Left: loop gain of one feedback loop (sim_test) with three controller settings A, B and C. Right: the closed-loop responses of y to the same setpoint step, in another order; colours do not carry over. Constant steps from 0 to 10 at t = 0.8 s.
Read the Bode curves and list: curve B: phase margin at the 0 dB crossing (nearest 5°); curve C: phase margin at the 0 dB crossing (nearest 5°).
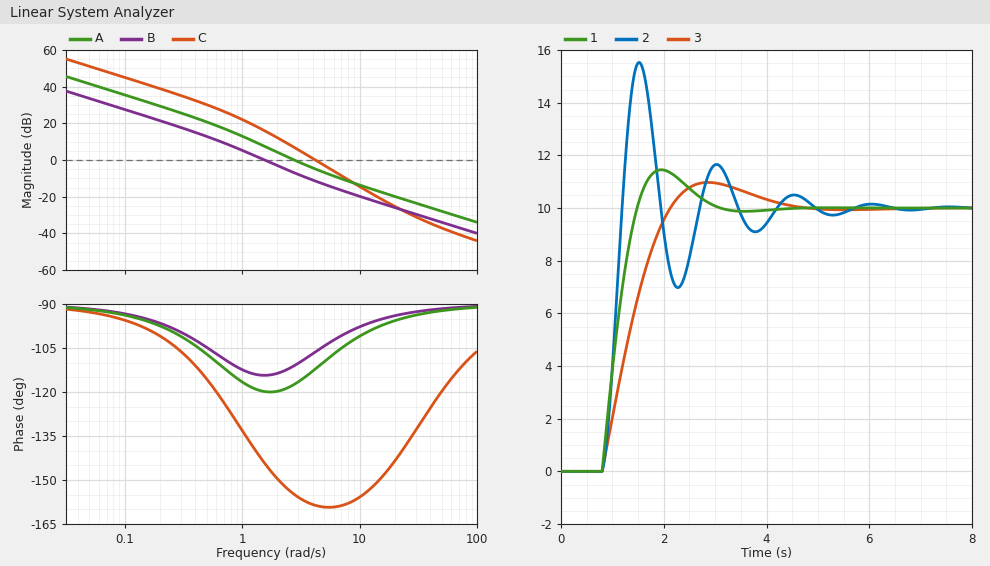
65°
20°
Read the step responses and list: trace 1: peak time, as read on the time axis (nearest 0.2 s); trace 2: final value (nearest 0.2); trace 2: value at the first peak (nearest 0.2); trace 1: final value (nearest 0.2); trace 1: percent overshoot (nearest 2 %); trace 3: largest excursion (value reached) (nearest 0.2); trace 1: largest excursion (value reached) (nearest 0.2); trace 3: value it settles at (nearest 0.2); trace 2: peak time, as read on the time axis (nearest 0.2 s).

2.0 s
10.0
15.6
10.0
14 %
11.0
11.4
10.0
1.6 s
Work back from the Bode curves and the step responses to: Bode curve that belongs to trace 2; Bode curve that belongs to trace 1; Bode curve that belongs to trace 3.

C
A
B
